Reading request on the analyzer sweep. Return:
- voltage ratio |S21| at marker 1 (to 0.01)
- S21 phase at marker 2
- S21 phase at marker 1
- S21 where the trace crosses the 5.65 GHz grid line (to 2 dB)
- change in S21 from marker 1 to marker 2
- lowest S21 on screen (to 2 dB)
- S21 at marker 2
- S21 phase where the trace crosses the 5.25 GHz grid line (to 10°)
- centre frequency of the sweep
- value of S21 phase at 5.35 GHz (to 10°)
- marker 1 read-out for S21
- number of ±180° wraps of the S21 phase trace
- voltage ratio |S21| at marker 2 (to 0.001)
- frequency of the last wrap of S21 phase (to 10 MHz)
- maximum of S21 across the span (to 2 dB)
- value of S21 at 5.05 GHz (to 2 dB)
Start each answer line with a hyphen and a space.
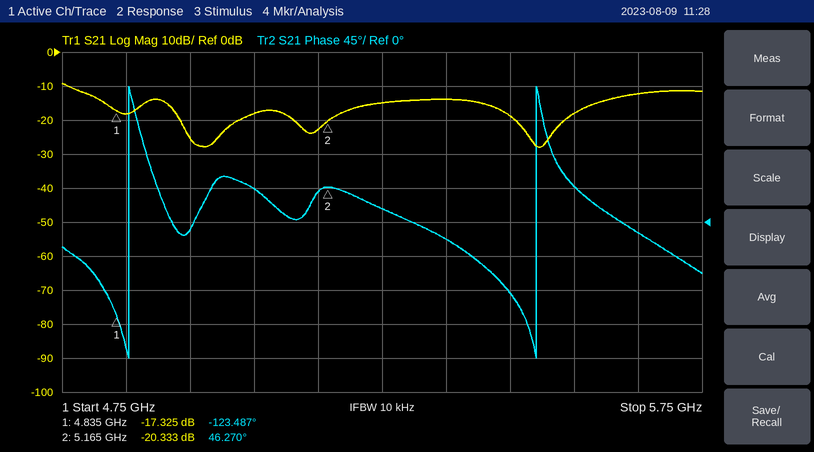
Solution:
- 0.14
- 46.270°
- -123.487°
- -12 dB
- -3.008 dB
- -28 dB
- -20.333 dB
- 20°
- 5.25 GHz
- -20°
- -17.325 dB
- 2
- 0.096
- 5.49 GHz
- -10 dB
- -18 dB
